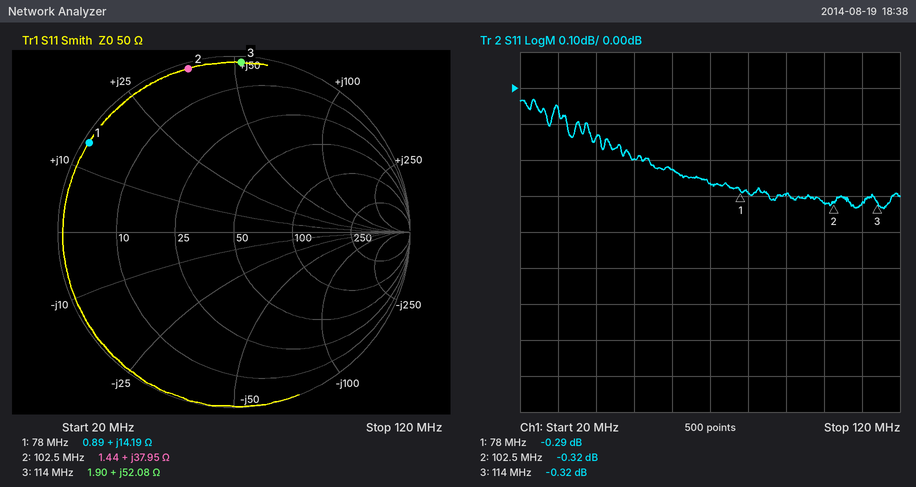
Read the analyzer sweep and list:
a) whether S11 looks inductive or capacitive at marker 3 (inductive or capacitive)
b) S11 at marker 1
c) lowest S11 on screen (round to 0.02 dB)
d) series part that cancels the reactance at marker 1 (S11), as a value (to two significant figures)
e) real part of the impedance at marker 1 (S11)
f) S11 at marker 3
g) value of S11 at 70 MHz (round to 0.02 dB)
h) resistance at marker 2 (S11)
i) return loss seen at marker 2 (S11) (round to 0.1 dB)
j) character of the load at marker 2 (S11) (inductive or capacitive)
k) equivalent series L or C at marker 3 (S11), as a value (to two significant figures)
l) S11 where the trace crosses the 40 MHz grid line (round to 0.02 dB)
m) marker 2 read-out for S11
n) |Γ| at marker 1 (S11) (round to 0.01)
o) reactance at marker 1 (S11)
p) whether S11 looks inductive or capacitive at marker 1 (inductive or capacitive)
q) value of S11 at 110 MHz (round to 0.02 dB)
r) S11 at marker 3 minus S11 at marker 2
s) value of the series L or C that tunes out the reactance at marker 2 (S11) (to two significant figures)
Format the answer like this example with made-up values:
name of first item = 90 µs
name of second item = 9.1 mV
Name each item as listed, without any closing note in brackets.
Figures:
whether S11 looks inductive or capacitive at marker 3 = inductive
S11 at marker 1 = -0.29 dB
lowest S11 on screen = -0.34 dB
series part that cancels the reactance at marker 1 (S11), as a value = 140 pF
real part of the impedance at marker 1 = 0.89 Ω
S11 at marker 3 = -0.32 dB
value of S11 at 70 MHz = -0.26 dB
resistance at marker 2 = 1.44 Ω
return loss seen at marker 2 (S11) = 0.3 dB
character of the load at marker 2 (S11) = inductive
equivalent series L or C at marker 3 (S11), as a value = 73 nH
S11 where the trace crosses the 40 MHz grid line = -0.14 dB
marker 2 read-out for S11 = -0.32 dB
|Γ| at marker 1 (S11) = 0.97
reactance at marker 1 = +14.19 Ω
whether S11 looks inductive or capacitive at marker 1 = inductive
value of S11 at 110 MHz = -0.32 dB
S11 at marker 3 minus S11 at marker 2 = 0.00 dB
value of the series L or C that tunes out the reactance at marker 2 (S11) = 41 pF
